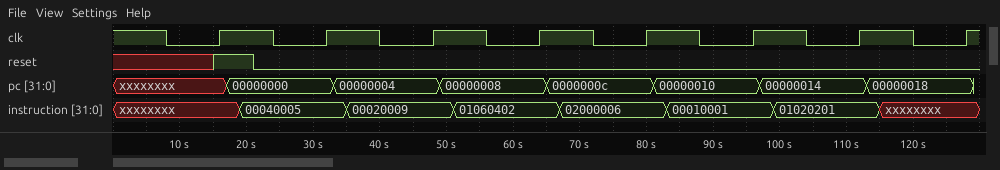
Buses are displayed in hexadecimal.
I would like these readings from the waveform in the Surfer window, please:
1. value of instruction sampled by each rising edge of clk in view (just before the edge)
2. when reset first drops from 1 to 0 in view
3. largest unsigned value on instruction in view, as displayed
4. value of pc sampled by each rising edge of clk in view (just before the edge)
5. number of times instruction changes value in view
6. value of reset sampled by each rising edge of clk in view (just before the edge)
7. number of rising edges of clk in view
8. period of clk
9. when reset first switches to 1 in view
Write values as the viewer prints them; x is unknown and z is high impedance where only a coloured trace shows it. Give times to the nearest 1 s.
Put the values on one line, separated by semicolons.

xxxxxxxx, 00040005, 00020009, 01060402, 02000006, 00010001, 01020201, xxxxxxxx; 21 s; 02000006; xxxxxxxx, 00000000, 00000004, 00000008, 0000000c, 00000010, 00000014, 00000018; 7; 1 0 0 0 0 0 0 0; 8; 16 s; 15 s
